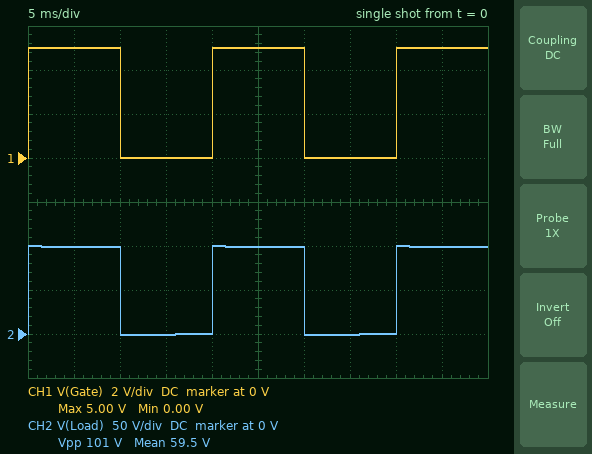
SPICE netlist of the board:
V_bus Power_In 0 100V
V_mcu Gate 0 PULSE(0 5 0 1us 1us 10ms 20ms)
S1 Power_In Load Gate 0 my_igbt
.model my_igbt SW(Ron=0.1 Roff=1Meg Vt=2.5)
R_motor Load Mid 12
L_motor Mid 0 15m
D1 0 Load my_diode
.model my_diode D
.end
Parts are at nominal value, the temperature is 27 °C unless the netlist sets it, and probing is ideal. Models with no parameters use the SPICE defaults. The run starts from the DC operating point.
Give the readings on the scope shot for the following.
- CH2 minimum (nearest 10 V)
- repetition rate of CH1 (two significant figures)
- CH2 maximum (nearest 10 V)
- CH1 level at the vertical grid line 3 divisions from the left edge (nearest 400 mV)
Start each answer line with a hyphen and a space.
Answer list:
- 0 V
- 50 Hz
- 100 V
- 0 V
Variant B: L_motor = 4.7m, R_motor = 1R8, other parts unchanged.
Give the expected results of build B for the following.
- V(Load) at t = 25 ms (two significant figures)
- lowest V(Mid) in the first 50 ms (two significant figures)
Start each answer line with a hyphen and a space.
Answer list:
- 95 V
- -94 V
